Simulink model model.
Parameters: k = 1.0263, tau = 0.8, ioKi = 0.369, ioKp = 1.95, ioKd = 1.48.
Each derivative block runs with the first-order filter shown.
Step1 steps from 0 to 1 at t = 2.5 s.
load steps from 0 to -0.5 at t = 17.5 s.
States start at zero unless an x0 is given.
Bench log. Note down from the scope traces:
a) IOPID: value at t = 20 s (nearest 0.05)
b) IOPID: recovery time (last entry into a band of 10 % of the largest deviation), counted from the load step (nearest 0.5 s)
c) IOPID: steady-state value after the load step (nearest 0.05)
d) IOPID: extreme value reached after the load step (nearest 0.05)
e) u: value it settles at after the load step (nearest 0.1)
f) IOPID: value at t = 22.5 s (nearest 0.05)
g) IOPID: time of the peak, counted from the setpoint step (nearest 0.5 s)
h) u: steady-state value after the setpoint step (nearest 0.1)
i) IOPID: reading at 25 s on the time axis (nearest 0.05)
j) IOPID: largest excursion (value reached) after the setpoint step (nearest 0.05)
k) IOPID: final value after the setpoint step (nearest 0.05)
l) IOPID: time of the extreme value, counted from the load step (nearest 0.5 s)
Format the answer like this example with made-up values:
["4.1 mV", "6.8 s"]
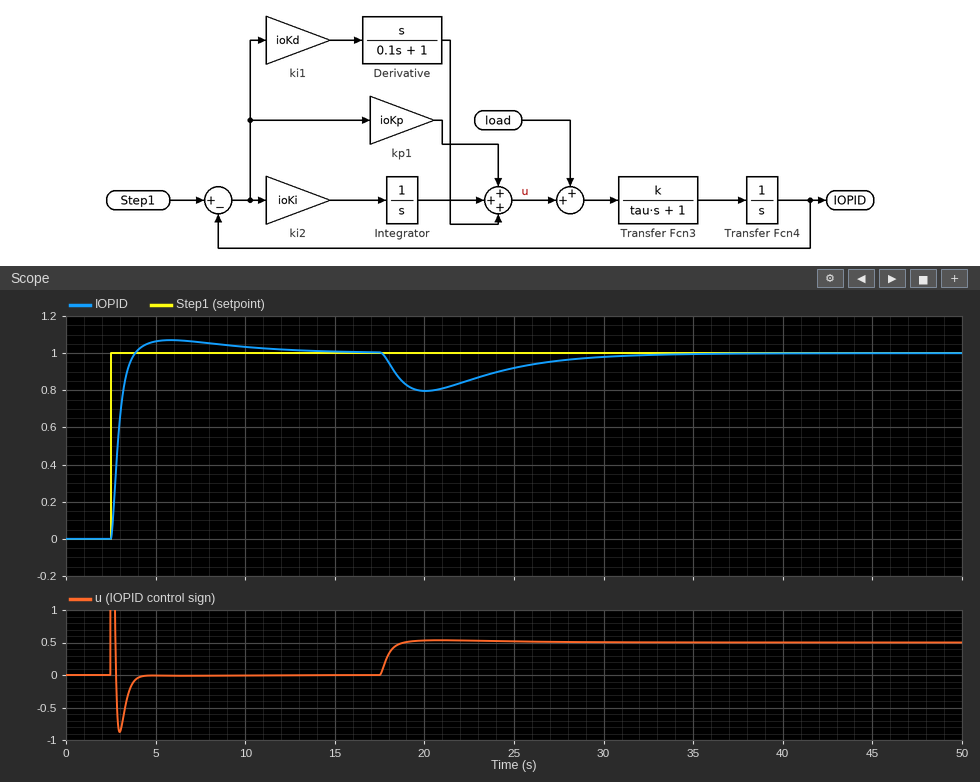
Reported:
["0.80", "12.5 s", "1.00", "0.80", "0.5", "0.85", "3.5 s", "0.0", "0.90", "1.05", "1.00", "2.5 s"]
